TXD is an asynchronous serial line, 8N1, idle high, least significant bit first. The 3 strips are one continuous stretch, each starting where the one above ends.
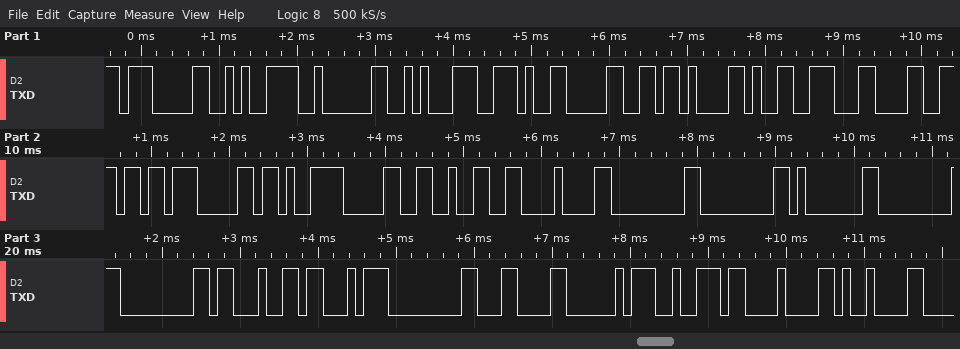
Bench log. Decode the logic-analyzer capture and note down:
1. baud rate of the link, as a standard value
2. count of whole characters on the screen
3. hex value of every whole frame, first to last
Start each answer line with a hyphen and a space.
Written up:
- 9600 baud
- 28
- 0x07 0xCA 0x02 0x8A 0x2E 0x30 0x0B 0x99 0x0C 0x6E 0x07 0xCB 0x30 0x32 0x08 0x00 0x00 0x01 0x00 0x00 0x23 0xA3 0x00 0x0C 0xA0 0x72 0x08 0x09
